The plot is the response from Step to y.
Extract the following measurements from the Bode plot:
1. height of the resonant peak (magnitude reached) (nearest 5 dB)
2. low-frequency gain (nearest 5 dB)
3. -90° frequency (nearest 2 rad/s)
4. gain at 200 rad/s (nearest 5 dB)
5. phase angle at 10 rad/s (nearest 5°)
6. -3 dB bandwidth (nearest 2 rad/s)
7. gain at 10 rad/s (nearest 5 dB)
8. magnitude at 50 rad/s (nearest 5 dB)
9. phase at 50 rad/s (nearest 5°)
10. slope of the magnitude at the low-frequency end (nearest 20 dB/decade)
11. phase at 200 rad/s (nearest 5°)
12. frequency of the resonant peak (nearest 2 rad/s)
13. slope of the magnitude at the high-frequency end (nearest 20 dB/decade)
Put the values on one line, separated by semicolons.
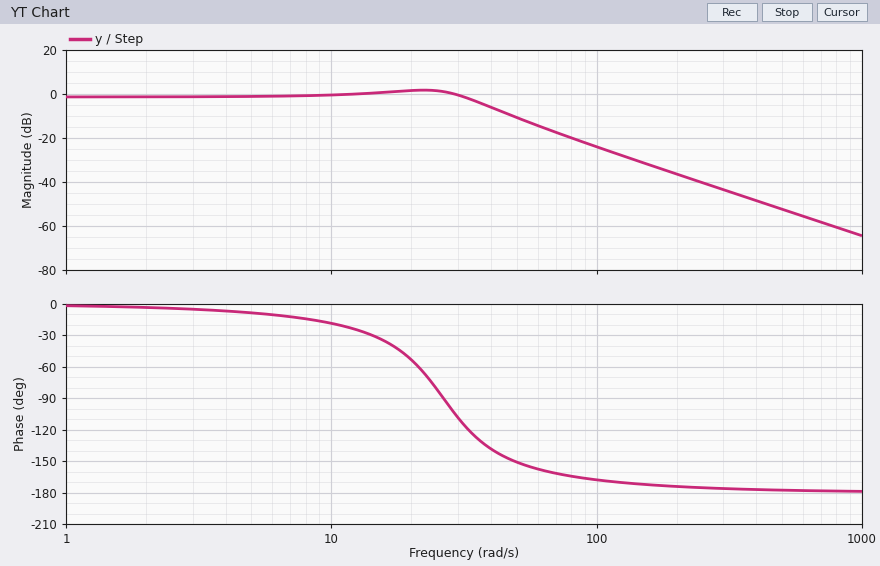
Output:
0 dB; 0 dB; 26 rad/s; -35 dB; -20°; 36 rad/s; 0 dB; -10 dB; -150°; 0 dB/decade; -175°; 22 rad/s; -40 dB/decade
